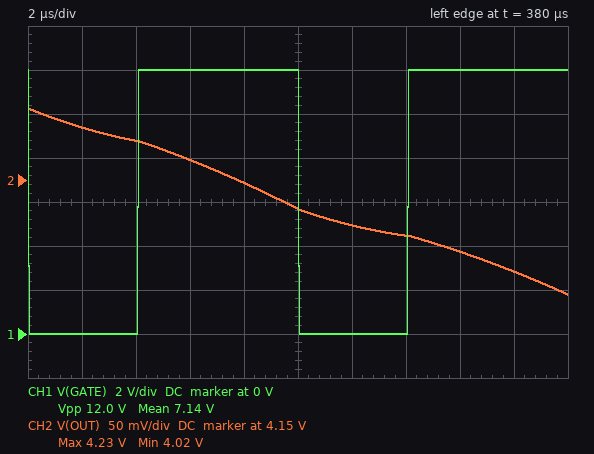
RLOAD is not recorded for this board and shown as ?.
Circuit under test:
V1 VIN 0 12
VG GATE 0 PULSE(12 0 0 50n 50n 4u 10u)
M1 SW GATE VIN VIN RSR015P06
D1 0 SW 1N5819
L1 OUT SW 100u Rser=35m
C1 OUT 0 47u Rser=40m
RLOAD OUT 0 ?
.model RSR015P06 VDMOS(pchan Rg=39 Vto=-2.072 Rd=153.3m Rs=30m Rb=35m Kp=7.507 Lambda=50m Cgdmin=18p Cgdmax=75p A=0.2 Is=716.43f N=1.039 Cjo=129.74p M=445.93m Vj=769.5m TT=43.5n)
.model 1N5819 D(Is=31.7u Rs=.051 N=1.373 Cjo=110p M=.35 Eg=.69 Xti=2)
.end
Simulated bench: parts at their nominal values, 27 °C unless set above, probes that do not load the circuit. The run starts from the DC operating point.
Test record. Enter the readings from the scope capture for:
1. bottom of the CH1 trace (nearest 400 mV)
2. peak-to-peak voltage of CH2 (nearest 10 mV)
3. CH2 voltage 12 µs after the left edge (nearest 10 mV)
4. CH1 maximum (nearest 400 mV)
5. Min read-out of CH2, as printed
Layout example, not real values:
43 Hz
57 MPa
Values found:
0 V
210 mV
4.10 V
12.0 V
4.02 V
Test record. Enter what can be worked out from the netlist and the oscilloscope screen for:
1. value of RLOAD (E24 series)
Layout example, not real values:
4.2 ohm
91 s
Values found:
5.1 Ω
